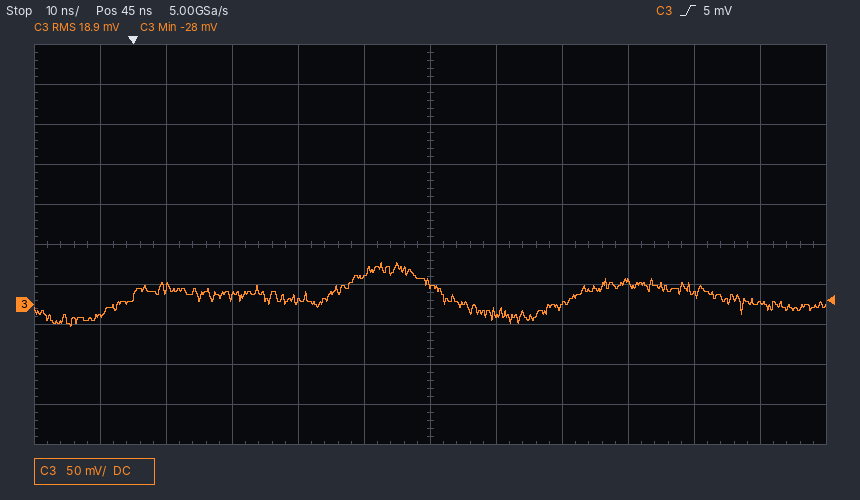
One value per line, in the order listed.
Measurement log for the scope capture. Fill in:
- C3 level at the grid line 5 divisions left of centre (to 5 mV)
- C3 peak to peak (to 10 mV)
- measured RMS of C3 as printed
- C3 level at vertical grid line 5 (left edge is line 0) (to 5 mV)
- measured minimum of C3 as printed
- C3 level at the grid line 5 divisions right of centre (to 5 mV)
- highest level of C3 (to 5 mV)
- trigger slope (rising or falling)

-15 mV
80 mV
18.9 mV
35 mV
-28 mV
0 mV
50 mV
rising
